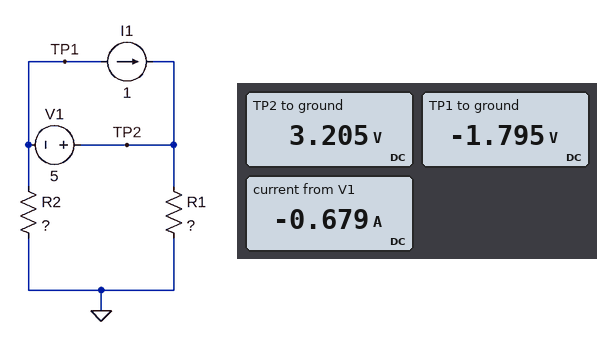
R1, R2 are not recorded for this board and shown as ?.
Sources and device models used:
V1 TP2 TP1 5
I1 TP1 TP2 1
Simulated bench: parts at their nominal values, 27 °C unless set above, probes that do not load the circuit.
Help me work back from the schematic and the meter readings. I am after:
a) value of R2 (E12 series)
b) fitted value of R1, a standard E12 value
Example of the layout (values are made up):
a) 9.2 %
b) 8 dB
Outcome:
a) 5.6 Ω
b) 10 Ω
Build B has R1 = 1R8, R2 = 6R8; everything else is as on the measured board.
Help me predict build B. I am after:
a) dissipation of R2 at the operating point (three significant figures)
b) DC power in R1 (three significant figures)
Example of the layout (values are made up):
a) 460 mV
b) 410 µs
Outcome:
a) 2.30 W
b) 608 mW
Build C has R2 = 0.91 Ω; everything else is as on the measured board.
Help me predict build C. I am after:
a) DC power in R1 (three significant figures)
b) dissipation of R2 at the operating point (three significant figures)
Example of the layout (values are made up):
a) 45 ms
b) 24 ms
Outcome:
a) 2.10 W
b) 191 mW
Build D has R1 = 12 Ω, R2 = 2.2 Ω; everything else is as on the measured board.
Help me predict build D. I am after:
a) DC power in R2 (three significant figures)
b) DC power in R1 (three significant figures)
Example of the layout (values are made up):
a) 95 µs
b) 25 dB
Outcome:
a) 273 mW
b) 1.49 W
